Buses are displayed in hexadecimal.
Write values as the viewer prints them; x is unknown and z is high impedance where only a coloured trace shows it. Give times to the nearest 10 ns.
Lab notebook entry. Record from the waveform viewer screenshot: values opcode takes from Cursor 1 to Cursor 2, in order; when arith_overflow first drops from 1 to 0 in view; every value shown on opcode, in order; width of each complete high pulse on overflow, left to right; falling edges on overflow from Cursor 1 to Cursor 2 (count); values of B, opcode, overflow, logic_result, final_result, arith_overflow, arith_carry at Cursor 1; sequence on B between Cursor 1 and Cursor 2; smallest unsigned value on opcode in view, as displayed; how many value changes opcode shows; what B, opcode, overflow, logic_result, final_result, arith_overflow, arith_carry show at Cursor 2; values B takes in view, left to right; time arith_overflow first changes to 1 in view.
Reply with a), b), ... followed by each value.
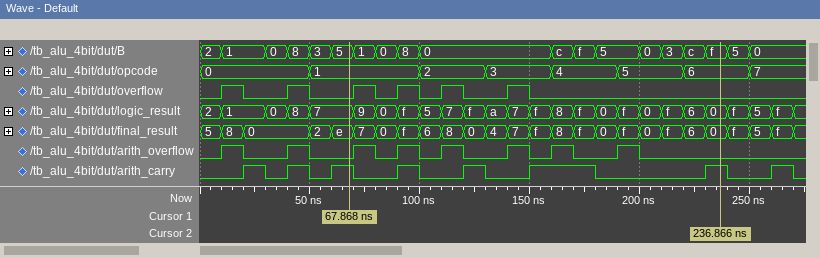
a) 1, 2, 3, 4, 5, 6
b) 20 ns
c) 0, 1, 2, 3, 4, 5, 6, 7
d) 10 ns, 10 ns, 10 ns, 10 ns, 10 ns, 10 ns
e) 4
f) B=5, opcode=1, overflow=0, logic_result=7, final_result=e, arith_overflow=0, arith_carry=1
g) 5, 1, 0, 8, 0, c, f, 5, 0, 3, c, f
h) 0
i) 7
j) B=f, opcode=6, overflow=0, logic_result=0, final_result=0, arith_overflow=0, arith_carry=1
k) 2, 1, 0, 8, 3, 5, 1, 0, 8, 0, c, f, 5, 0, 3, c, f, 5, 0
l) 10 ns
